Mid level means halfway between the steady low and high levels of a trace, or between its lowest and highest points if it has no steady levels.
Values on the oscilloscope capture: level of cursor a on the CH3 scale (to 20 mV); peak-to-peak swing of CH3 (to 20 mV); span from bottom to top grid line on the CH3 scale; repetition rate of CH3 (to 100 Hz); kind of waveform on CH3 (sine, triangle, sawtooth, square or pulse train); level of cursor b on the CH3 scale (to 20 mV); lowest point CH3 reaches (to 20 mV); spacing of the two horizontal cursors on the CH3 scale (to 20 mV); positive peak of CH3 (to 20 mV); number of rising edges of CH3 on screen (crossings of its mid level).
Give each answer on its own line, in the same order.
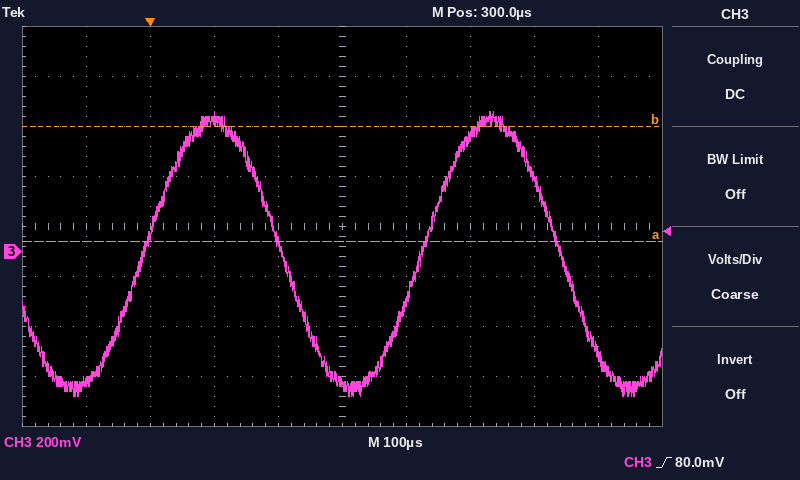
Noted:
40 mV
1.14 V
1.6 V
2.3 kHz
sine
500 mV
-580 mV
460 mV
560 mV
2
